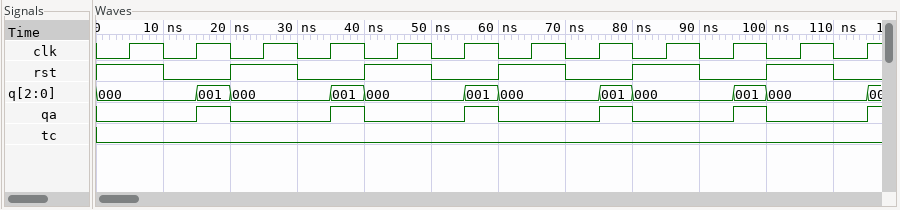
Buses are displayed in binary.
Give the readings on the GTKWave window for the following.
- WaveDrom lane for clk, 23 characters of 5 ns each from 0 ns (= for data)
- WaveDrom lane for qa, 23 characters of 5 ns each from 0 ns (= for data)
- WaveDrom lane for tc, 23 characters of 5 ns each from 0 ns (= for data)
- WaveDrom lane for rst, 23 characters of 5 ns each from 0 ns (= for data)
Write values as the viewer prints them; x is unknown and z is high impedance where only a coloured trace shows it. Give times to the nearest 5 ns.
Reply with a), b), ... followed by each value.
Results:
a) {name: 'clk', wave: '01010101010101010101010'}
b) {name: 'qa', wave: '0..10..10..10..10..10..'}
c) {name: 'tc', wave: '0......................'}
d) {name: 'rst', wave: '1.0.1.0.1.0.1.0.1.0.1.0'}
